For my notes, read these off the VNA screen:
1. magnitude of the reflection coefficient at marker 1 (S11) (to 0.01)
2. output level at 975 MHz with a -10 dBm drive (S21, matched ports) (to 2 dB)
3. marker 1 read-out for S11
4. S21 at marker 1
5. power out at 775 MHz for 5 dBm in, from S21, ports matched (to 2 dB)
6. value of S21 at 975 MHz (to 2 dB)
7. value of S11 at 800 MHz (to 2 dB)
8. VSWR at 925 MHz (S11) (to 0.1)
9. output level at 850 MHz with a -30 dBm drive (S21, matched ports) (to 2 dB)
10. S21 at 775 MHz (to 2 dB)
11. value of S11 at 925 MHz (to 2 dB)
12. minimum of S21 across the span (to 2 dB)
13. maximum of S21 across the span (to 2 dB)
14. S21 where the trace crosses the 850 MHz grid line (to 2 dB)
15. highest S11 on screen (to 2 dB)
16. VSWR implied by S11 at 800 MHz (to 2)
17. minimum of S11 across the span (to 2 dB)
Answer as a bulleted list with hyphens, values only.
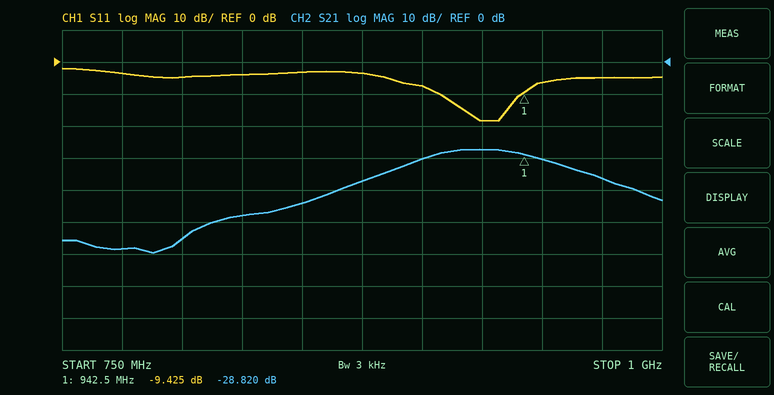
- 0.34
- -46 dBm
- -9.425 dB
- -28.820 dB
- -54 dBm
- -36 dB
- -4 dB
- 1.3
- -74 dBm
- -58 dB
- -18 dB
- -60 dB
- -28 dB
- -44 dB
- -2 dB
- 4
- -18 dB
